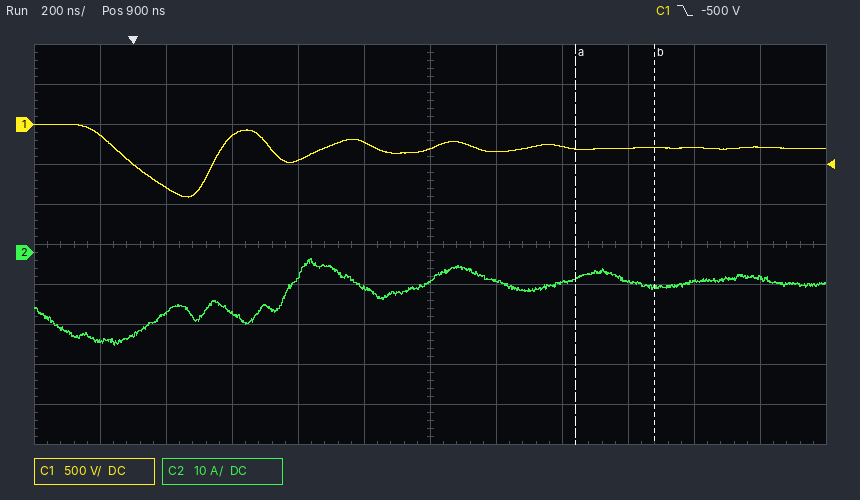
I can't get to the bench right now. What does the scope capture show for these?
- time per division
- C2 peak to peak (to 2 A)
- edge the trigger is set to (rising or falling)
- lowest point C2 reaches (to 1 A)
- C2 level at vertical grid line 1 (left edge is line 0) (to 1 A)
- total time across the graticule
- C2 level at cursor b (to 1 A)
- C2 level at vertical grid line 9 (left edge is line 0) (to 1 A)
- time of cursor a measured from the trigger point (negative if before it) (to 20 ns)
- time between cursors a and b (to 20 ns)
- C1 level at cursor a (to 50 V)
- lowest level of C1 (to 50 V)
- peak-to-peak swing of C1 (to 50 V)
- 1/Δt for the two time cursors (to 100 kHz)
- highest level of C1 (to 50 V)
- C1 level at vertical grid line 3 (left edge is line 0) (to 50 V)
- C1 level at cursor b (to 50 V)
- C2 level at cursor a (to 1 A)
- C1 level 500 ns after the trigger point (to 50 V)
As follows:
200 ns
22 A
falling
-23 A
-22 A
2.4 µs
-9 A
-7 A
+1.34 µs
240 ns
-300 V
-900 V
900 V
4.2 MHz
0 V
-150 V
-300 V
-7 A
-450 V
